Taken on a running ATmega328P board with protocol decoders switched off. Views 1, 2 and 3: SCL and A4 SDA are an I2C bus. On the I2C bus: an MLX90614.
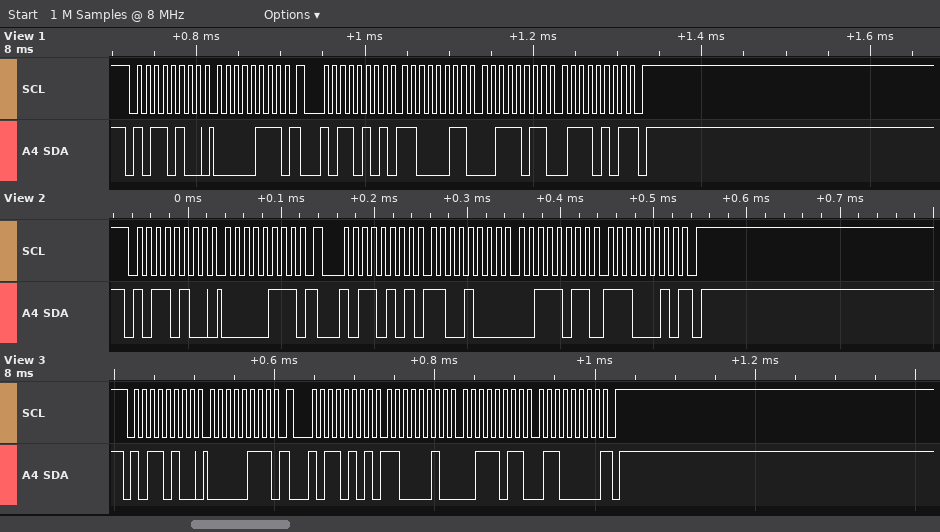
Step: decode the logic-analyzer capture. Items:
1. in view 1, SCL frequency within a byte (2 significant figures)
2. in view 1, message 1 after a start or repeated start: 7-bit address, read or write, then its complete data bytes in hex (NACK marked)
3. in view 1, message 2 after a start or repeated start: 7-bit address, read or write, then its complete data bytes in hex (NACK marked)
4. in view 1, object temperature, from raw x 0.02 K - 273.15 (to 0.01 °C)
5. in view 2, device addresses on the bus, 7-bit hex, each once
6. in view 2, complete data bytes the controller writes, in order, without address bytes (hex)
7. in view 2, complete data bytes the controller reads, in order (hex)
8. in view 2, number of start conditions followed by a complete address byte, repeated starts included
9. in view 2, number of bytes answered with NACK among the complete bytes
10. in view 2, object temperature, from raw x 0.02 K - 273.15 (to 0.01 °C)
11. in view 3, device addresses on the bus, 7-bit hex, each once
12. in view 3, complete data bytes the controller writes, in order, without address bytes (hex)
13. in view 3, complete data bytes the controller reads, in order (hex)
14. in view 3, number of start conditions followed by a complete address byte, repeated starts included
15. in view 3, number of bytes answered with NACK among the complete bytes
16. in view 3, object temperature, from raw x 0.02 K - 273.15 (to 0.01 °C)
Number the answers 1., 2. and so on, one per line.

1. 100 kHz
2. 0x5A write: 07
3. 0x5A read: C3 3B 75 NACK
4. 32.83 °C
5. 0x5A
6. 07
7. C8 3B E2
8. 2
9. 1
10. 32.93 °C
11. 0x5A
12. 07
13. C2 3B 60
14. 2
15. 1
16. 32.81 °C
